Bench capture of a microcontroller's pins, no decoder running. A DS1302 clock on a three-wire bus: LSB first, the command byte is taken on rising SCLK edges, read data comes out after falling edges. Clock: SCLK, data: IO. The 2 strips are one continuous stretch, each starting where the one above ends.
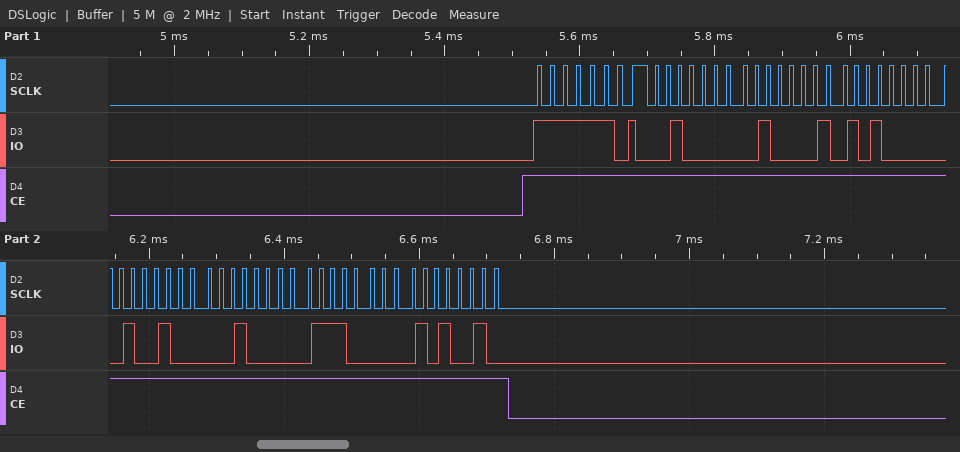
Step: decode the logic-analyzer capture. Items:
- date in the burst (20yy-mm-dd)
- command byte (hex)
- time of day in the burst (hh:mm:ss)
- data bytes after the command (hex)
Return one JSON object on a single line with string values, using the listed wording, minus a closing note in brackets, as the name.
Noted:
{"date in the burst": "2025-04-12", "command byte": "0xBF", "time of day in the burst": "05:42:04", "data bytes after the command": "04 42 05 12 04 07 25"}
